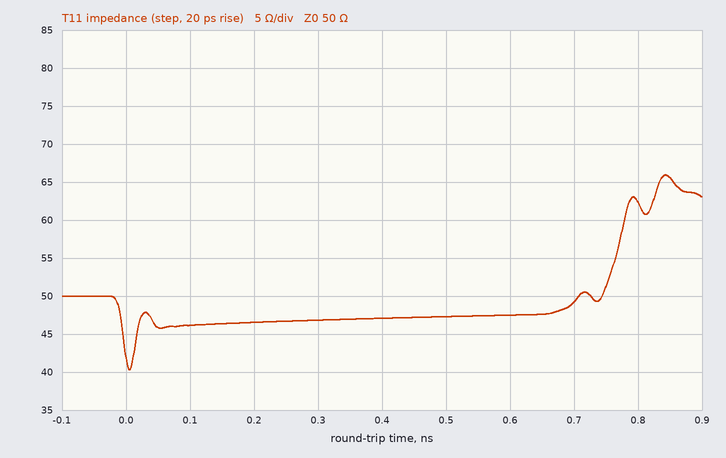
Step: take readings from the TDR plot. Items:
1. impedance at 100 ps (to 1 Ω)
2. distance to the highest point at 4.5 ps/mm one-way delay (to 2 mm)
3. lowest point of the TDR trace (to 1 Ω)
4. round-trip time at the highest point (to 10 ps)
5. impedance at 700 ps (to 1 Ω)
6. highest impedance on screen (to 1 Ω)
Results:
46 Ω
94 mm
40 Ω
840 ps
49 Ω
66 Ω
